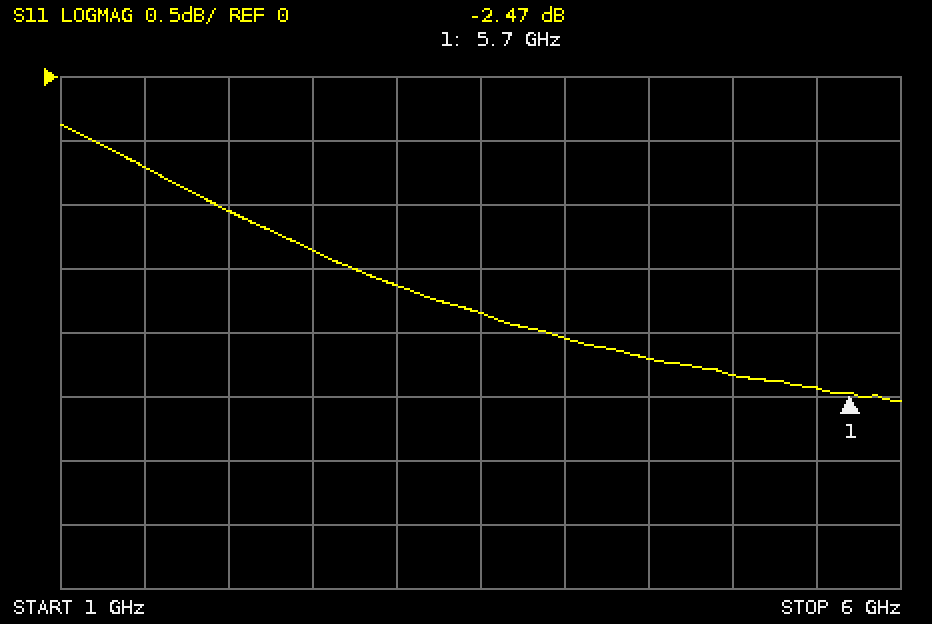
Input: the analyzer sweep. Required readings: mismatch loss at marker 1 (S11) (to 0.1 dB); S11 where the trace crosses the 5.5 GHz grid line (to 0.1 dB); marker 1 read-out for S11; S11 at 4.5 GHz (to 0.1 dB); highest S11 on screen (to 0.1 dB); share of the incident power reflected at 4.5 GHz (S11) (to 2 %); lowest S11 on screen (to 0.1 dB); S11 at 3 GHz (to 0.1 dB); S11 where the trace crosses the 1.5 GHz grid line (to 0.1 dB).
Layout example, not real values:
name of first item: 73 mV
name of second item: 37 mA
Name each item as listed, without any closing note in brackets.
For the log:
mismatch loss at marker 1 (S11): 3.6 dB
S11 where the trace crosses the 5.5 GHz grid line: -2.4 dB
marker 1 read-out for S11: -2.47 dB
S11 at 4.5 GHz: -2.2 dB
highest S11 on screen: -0.4 dB
share of the incident power reflected at 4.5 GHz (S11): 60 %
lowest S11 on screen: -2.5 dB
S11 at 3 GHz: -1.6 dB
S11 where the trace crosses the 1.5 GHz grid line: -0.7 dB
